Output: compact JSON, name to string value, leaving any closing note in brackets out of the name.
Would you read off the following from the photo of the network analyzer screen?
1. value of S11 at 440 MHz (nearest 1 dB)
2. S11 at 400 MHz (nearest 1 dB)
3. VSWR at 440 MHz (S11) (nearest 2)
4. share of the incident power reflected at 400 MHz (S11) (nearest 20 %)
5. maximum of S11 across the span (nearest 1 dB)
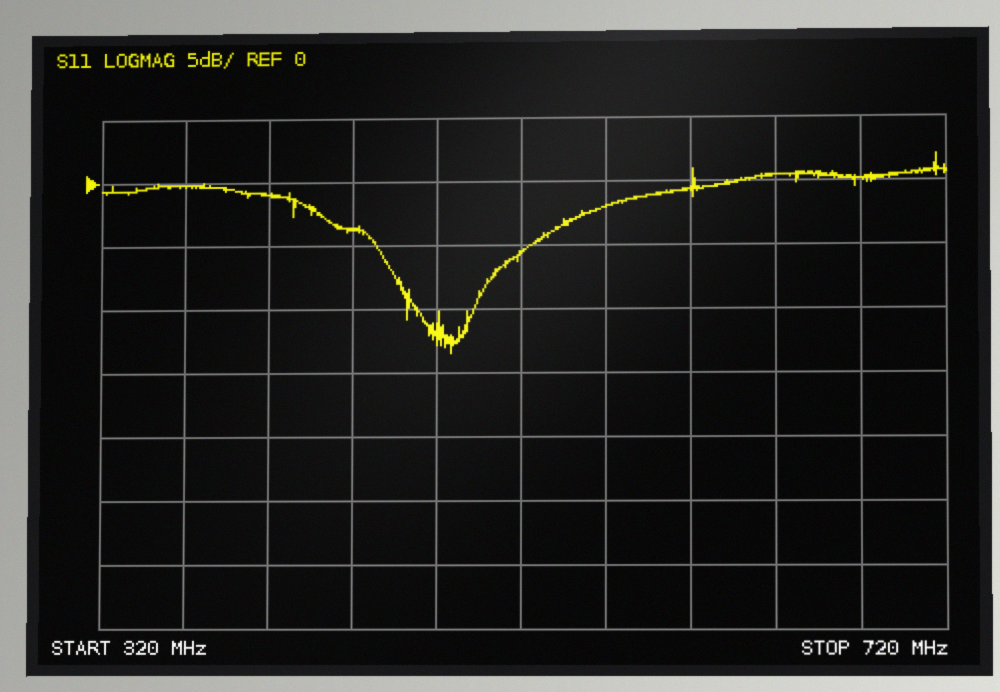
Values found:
{"value of S11 at 440 MHz": "-4 dB", "S11 at 400 MHz": "-1 dB", "VSWR at 440 MHz (S11)": "4", "share of the incident power reflected at 400 MHz (S11)": "80 %", "maximum of S11 across the span": "2 dB"}
